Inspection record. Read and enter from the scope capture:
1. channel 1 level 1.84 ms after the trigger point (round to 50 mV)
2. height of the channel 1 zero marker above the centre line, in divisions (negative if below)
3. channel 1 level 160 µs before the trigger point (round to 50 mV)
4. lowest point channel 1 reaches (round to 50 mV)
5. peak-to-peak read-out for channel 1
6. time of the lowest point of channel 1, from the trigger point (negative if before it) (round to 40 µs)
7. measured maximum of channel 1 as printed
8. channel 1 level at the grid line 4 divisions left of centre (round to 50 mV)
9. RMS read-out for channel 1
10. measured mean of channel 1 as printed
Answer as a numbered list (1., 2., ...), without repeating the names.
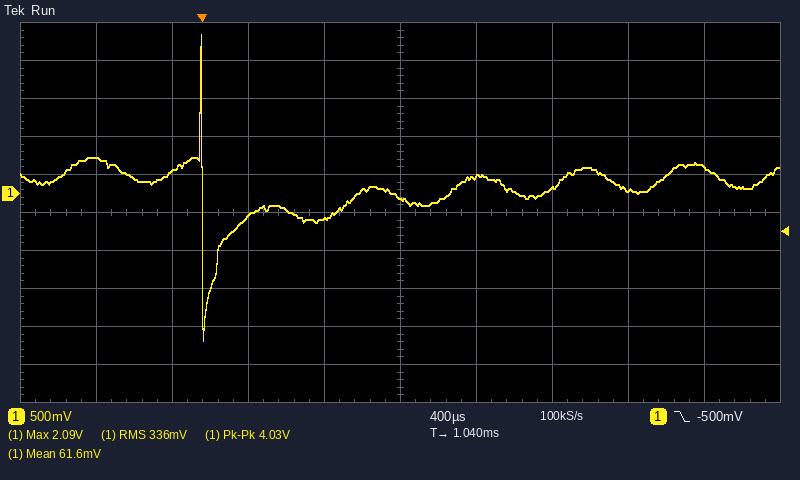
1. 50 mV
2. +0.5 div
3. 300 mV
4. -1.95 V
5. 4.03 V
6. 0 µs
7. 2.09 V
8. 450 mV
9. 336 mV
10. 61.6 mV
